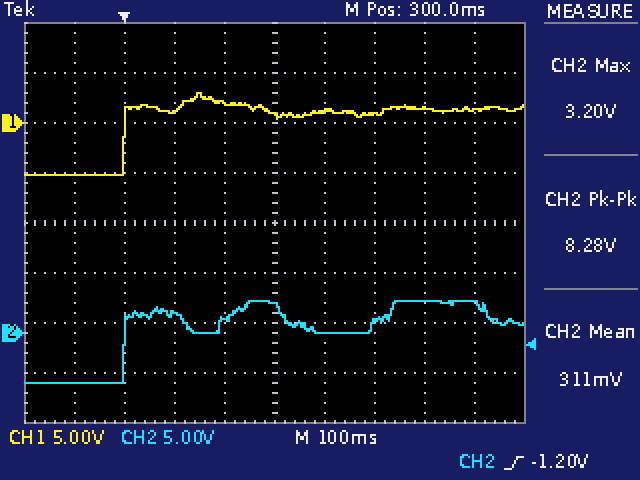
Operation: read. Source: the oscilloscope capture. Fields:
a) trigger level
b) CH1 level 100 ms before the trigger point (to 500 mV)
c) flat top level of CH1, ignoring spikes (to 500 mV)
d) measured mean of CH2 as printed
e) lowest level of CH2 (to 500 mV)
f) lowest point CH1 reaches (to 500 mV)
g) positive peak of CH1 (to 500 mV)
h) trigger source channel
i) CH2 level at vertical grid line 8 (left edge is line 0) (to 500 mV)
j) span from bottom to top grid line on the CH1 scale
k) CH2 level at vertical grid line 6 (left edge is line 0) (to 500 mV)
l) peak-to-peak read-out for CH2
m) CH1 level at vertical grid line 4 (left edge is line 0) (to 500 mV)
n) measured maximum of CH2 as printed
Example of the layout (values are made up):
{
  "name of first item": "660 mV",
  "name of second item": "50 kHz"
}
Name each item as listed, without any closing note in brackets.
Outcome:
{
  "trigger level": "-1.20 V",
  "CH1 level 100 ms before the trigger point": "-5.0 V",
  "flat top level of CH1, ignoring spikes": "1.5 V",
  "measured mean of CH2 as printed": "311 mV",
  "lowest level of CH2": "-5.0 V",
  "lowest point CH1 reaches": "-5.0 V",
  "positive peak of CH1": "3.0 V",
  "trigger source channel": "CH2",
  "CH2 level at vertical grid line 8 (left edge is line 0)": "3.0 V",
  "span from bottom to top grid line on the CH1 scale": "40 V",
  "CH2 level at vertical grid line 6 (left edge is line 0)": "0.0 V",
  "peak-to-peak read-out for CH2": "8.28 V",
  "CH1 level at vertical grid line 4 (left edge is line 0)": "2.0 V",
  "measured maximum of CH2 as printed": "3.20 V"
}
